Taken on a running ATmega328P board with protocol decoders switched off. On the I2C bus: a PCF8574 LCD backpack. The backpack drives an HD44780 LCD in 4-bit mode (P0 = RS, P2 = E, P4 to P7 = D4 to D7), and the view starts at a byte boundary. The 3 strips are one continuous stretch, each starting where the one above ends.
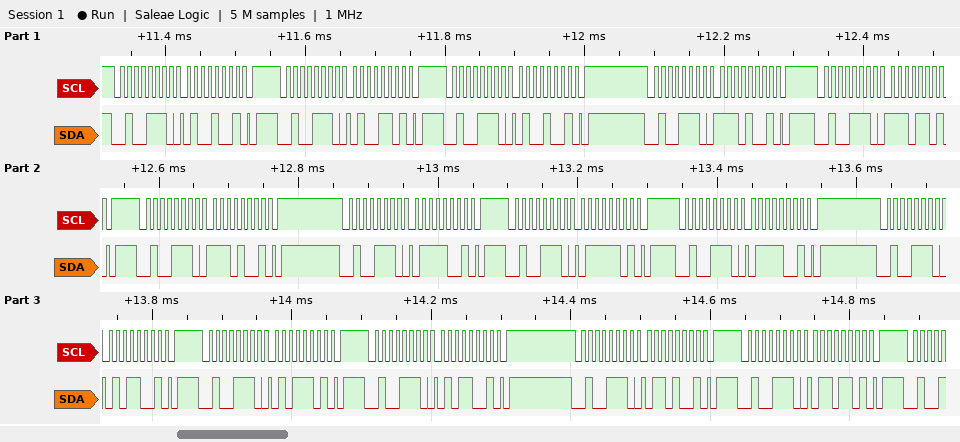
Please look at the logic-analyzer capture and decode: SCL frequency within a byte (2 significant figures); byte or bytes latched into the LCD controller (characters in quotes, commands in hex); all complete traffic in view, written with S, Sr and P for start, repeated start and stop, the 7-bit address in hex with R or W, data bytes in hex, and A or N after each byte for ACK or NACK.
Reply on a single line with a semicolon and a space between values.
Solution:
100 kHz; 'N' 'u'; S 27W A 49 A P S 27W A 4D A P S 27W A 49 A P S 27W A E9 A P S 27W A ED A P S 27W A E9 A P S 27W A 79 A P S 27W A 7D A P S 27W A 79 A P S 27W A 59 A P S 27W A 5D A P S 27W A 59 A P S 27W A 69 A P S 27W A 6D A P
